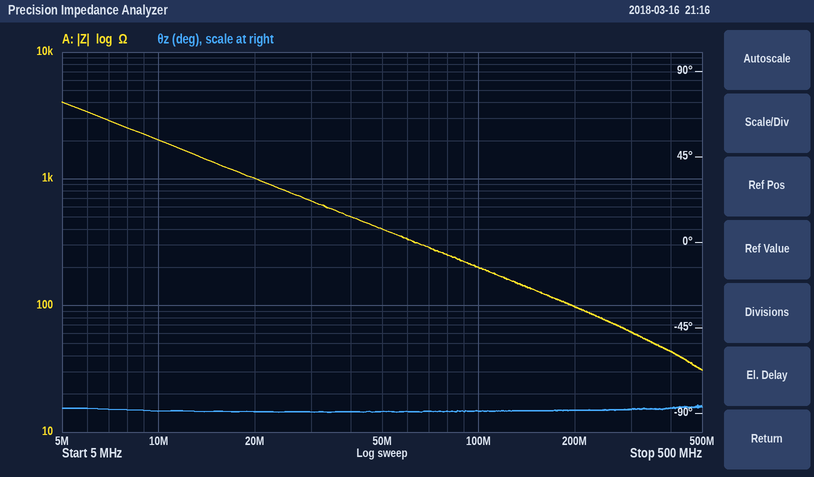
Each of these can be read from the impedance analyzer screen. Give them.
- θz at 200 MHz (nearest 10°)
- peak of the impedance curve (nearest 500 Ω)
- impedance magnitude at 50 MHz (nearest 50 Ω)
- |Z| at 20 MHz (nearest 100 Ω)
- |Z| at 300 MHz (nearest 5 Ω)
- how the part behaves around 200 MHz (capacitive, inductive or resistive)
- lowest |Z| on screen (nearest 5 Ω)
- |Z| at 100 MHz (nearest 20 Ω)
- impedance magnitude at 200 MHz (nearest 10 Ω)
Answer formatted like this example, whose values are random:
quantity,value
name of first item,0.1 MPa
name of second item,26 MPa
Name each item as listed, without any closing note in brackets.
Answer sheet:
quantity,value
θz at 200 MHz,-90°
peak of the impedance curve,4.0 kΩ
impedance magnitude at 50 MHz,400 Ω
|Z| at 20 MHz,1.0 kΩ
|Z| at 300 MHz,60 Ω
how the part behaves around 200 MHz,capacitive
lowest |Z| on screen,30 Ω
|Z| at 100 MHz,200 Ω
impedance magnitude at 200 MHz,100 Ω
